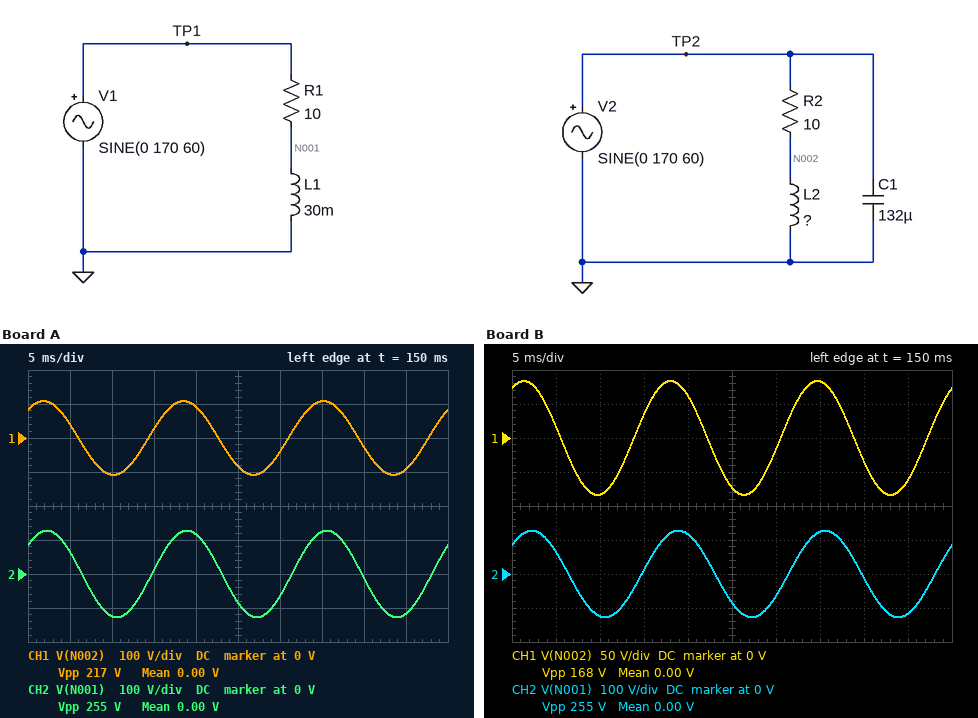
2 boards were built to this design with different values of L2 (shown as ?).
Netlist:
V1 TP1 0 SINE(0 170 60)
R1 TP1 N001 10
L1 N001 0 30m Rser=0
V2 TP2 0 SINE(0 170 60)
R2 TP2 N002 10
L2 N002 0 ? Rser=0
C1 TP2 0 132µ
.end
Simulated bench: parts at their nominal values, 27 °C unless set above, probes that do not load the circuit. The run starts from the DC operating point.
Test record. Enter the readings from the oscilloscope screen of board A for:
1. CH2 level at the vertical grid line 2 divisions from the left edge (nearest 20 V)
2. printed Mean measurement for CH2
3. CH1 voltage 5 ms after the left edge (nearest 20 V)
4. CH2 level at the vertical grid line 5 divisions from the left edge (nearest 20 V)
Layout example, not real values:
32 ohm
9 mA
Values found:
-120 V
0.00 V
40 V
-80 V
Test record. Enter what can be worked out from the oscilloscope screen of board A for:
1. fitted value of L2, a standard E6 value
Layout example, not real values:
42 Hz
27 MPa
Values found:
22 mH
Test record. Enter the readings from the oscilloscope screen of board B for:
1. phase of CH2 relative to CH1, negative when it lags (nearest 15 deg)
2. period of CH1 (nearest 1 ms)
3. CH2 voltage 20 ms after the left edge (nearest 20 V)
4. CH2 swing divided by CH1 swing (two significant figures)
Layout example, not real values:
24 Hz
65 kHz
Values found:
-15 deg
17 ms
120 V
1.5
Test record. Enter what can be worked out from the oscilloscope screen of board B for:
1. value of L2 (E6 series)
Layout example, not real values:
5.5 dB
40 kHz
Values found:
15 mH
